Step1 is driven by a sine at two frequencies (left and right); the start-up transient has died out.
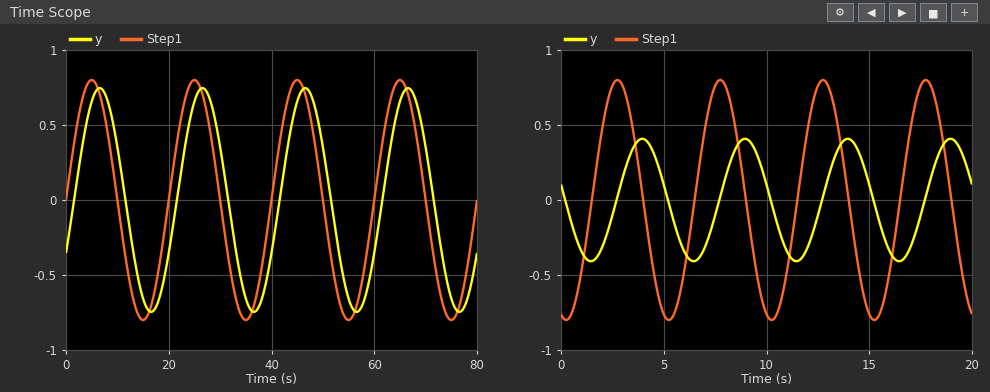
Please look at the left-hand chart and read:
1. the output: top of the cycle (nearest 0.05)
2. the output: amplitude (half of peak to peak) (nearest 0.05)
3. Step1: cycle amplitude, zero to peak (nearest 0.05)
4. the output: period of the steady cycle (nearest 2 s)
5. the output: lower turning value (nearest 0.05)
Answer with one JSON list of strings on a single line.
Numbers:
["0.75", "0.75", "0.80", "20 s", "-0.75"]
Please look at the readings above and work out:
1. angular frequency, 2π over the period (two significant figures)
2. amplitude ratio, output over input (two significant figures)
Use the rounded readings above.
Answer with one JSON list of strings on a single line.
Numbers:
["0.31 rad/s", "0.94"]
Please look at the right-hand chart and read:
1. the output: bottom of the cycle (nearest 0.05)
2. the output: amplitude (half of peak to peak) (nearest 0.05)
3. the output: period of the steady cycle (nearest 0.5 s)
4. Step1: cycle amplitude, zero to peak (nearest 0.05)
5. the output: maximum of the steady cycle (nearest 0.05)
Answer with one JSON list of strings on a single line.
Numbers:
["-0.40", "0.40", "5.0 s", "0.80", "0.40"]
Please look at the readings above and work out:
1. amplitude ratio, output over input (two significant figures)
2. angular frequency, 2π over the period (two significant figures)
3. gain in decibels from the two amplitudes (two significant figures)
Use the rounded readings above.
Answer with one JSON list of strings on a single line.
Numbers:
["0.50", "1.3 rad/s", "-6.0 dB"]
